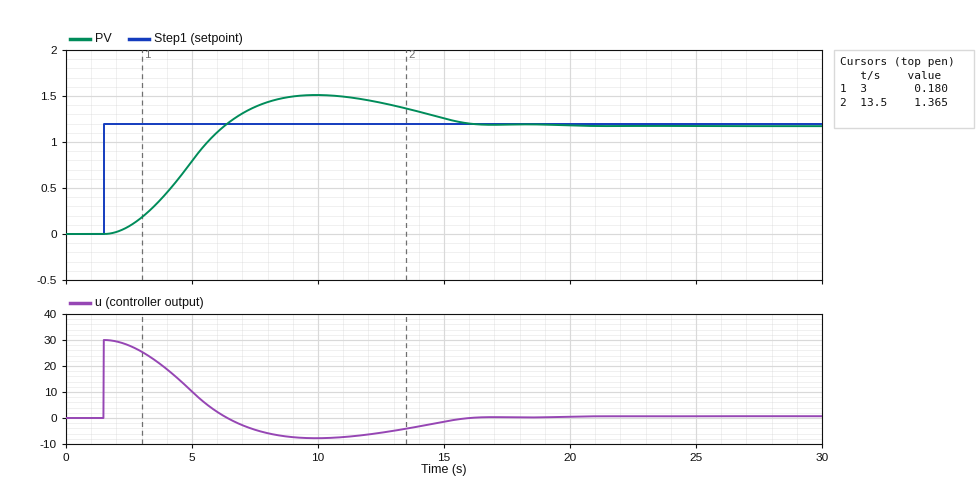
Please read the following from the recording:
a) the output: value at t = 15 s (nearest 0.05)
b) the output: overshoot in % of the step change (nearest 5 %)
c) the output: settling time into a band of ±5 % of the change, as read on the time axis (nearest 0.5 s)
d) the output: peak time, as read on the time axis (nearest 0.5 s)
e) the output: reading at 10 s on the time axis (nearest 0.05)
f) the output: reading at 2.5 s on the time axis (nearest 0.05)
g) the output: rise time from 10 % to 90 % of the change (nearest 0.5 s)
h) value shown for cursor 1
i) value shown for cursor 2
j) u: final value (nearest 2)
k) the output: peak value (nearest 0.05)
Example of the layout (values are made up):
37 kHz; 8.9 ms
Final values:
1.25; 30 %; 15.5 s; 10.0 s; 1.50; 0.10; 3.0 s; 0.180; 1.365; 0; 1.50
